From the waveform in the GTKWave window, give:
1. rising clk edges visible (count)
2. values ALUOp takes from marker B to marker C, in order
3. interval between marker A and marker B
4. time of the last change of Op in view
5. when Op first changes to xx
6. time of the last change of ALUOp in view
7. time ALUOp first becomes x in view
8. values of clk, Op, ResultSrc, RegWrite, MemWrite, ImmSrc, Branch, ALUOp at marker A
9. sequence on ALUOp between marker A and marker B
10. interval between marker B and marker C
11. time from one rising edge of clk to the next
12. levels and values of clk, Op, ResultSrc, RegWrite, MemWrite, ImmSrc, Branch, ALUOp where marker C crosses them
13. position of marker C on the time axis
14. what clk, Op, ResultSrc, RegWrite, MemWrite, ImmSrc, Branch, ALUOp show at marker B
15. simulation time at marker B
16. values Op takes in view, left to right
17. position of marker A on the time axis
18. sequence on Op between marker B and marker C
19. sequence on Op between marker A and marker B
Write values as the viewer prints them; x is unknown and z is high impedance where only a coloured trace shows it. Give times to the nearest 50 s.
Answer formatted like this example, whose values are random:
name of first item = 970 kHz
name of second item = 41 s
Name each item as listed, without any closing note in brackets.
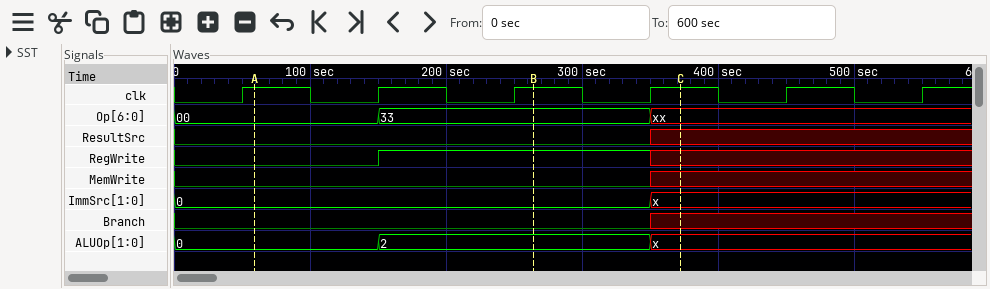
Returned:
rising clk edges visible = 6
values ALUOp takes from marker B to marker C, in order = 2, x
interval between marker A and marker B = 200 s
time of the last change of Op in view = 350 s
when Op first changes to xx = 350 s
time of the last change of ALUOp in view = 350 s
time ALUOp first becomes x in view = 350 s
values of clk, Op, ResultSrc, RegWrite, MemWrite, ImmSrc, Branch, ALUOp at marker A = clk=1, Op=00, ResultSrc=0, RegWrite=0, MemWrite=0, ImmSrc=0, Branch=0, ALUOp=0
sequence on ALUOp between marker A and marker B = 0, 2
interval between marker B and marker C = 100 s
time from one rising edge of clk to the next = 100 s
levels and values of clk, Op, ResultSrc, RegWrite, MemWrite, ImmSrc, Branch, ALUOp where marker C crosses them = clk=1, Op=xx, ResultSrc=x, RegWrite=x, MemWrite=x, ImmSrc=x, Branch=x, ALUOp=x
position of marker C on the time axis = 350 s
what clk, Op, ResultSrc, RegWrite, MemWrite, ImmSrc, Branch, ALUOp show at marker B = clk=1, Op=33, ResultSrc=0, RegWrite=1, MemWrite=0, ImmSrc=0, Branch=0, ALUOp=2
simulation time at marker B = 250 s
values Op takes in view, left to right = 00, 33, xx
position of marker A on the time axis = 50 s
sequence on Op between marker B and marker C = 33, xx
sequence on Op between marker A and marker B = 00, 33
